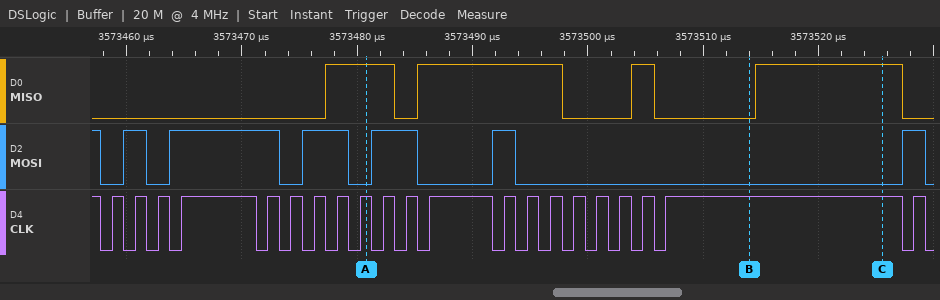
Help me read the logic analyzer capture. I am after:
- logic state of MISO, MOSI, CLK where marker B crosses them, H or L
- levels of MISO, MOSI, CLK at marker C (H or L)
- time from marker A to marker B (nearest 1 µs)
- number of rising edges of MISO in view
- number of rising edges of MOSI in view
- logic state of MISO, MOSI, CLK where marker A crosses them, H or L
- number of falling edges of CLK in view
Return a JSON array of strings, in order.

["MISO=L, MOSI=L, CLK=H", "MISO=H, MOSI=L, CLK=H", "33 µs", "4", "6", "MISO=H, MOSI=L, CLK=H", "22"]
